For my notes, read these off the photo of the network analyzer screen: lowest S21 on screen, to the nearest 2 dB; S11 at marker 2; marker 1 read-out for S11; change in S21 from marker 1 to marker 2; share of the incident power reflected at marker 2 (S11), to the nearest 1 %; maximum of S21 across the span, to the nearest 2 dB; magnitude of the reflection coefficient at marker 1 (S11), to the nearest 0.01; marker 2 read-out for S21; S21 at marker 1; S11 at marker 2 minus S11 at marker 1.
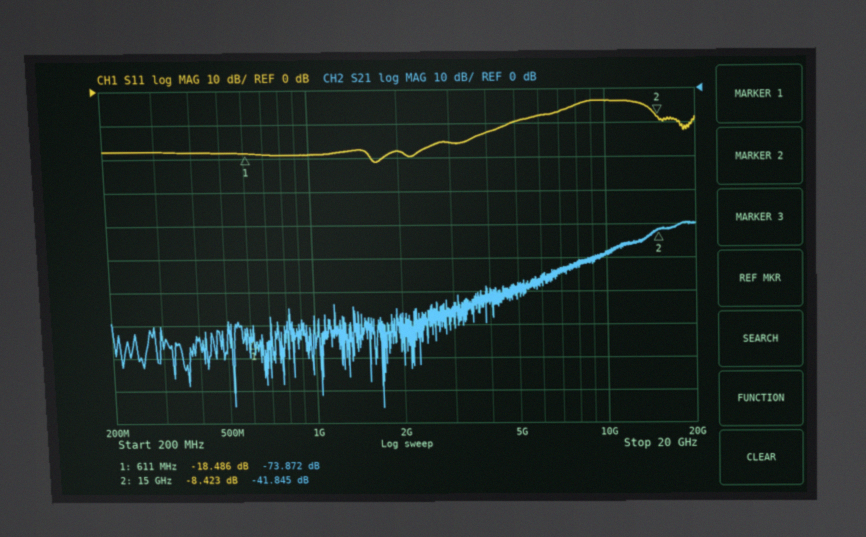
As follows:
-96 dB
-8.423 dB
-18.486 dB
32.027 dB
14 %
-40 dB
0.12
-41.845 dB
-73.872 dB
10.063 dB
